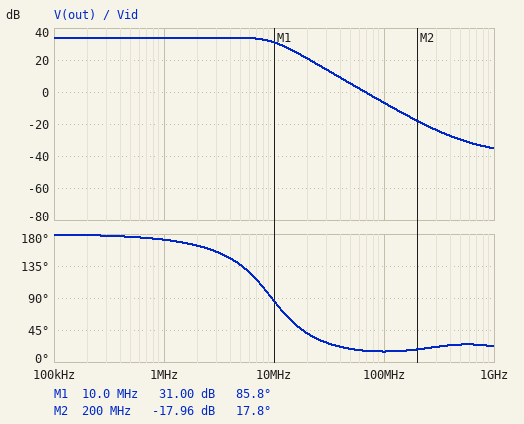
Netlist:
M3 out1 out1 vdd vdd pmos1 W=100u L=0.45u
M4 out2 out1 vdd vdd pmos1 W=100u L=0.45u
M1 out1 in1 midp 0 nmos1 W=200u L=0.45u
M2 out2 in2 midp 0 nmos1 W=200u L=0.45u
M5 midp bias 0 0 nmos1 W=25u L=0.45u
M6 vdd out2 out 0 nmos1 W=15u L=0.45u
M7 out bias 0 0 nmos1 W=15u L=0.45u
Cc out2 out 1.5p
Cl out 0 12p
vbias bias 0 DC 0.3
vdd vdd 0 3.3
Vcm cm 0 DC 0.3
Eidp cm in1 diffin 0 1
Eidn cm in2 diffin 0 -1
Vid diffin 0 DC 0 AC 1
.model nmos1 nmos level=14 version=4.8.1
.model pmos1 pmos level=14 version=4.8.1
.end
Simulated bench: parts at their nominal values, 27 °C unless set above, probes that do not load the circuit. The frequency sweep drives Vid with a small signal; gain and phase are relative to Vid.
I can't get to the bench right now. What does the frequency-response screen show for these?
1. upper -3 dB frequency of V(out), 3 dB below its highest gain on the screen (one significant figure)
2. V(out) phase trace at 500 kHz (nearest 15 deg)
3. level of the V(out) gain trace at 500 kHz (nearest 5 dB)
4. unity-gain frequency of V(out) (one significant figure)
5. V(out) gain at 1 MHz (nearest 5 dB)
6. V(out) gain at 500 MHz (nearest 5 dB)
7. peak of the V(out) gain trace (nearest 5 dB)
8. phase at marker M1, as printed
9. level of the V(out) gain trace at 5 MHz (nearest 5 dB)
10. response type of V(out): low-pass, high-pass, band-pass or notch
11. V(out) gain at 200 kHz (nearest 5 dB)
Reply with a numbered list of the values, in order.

1. 10 MHz
2. 180 deg
3. 35 dB
4. 70 MHz
5. 35 dB
6. -30 dB
7. 35 dB
8. 85.8 deg
9. 35 dB
10. low-pass
11. 35 dB
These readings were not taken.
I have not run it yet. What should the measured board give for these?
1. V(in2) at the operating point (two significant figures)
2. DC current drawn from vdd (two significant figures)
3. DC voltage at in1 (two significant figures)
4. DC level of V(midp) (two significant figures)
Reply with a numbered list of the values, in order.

1. 300 mV
2. 190 µA
3. 300 mV
4. 130 mV
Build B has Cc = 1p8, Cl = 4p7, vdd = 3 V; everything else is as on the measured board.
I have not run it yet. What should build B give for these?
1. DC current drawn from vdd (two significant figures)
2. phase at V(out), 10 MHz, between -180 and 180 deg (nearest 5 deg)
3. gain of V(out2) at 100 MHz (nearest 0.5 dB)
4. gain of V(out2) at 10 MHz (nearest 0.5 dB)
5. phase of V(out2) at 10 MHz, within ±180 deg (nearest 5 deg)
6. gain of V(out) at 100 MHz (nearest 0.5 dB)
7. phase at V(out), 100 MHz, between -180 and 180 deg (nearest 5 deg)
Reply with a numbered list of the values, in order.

1. 180 µA
2. 105 deg
3. 6.5 dB
4. 33.0 dB
5. 115 deg
6. -0.5 dB
7. 25 deg
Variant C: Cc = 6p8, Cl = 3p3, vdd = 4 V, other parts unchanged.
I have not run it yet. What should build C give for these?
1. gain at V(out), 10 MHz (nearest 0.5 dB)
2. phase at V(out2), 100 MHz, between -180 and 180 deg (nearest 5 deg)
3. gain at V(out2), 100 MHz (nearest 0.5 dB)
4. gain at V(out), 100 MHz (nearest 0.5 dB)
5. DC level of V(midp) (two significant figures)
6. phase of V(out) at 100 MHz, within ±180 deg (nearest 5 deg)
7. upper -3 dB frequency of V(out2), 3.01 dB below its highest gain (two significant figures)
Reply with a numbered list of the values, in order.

1. 29.0 dB
2. 60 deg
3. 3.5 dB
4. 0.5 dB
5. 150 mV
6. 55 deg
7. 9.6 MHz
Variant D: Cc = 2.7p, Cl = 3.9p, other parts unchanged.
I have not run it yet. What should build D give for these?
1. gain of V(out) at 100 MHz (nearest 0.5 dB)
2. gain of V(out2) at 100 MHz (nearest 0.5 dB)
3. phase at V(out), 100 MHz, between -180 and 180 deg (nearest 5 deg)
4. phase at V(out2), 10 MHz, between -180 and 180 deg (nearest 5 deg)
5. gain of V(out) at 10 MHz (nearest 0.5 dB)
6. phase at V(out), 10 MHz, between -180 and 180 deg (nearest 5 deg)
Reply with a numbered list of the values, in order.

1. 0 dB
2. 5.5 dB
3. 35 deg
4. 115 deg
5. 31.5 dB
6. 110 deg
